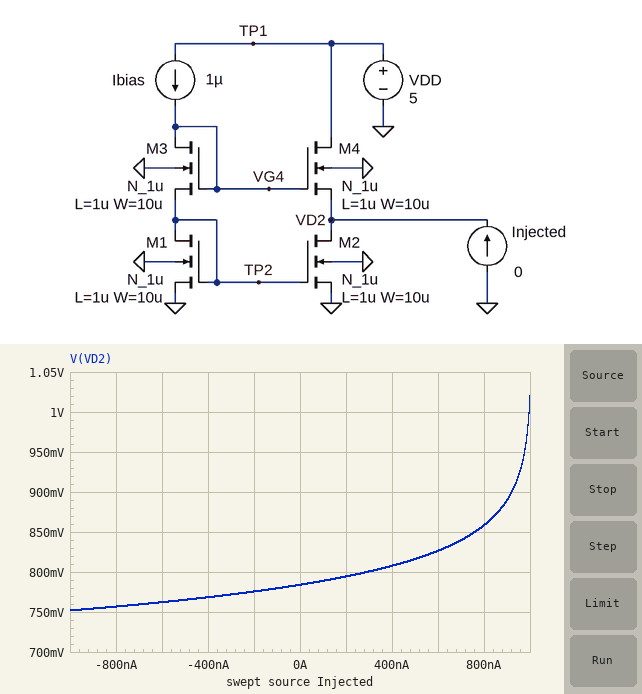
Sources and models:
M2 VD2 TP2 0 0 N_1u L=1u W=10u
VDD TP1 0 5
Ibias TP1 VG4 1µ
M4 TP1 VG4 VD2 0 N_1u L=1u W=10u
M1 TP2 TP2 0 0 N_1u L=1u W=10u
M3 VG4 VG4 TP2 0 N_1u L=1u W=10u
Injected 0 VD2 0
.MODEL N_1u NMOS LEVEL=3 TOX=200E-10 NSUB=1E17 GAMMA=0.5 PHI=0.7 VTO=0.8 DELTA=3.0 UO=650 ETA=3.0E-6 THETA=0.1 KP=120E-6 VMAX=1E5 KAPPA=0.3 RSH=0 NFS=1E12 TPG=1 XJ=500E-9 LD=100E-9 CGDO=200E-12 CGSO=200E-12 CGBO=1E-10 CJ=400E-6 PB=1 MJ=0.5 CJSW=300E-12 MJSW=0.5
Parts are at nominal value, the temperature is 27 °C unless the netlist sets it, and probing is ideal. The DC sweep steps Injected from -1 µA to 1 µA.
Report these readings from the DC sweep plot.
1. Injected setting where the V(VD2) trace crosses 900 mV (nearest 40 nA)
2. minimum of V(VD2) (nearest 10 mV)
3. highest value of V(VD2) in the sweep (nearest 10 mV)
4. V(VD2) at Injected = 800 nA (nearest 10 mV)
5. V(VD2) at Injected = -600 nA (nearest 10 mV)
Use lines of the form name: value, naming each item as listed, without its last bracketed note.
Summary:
Injected setting where the V(VD2) trace crosses 900 mV: 920 nA
minimum of V(VD2): 750 mV
highest value of V(VD2) in the sweep: 1.02 V
V(VD2) at Injected = 800 nA: 860 mV
V(VD2) at Injected = -600 nA: 760 mV
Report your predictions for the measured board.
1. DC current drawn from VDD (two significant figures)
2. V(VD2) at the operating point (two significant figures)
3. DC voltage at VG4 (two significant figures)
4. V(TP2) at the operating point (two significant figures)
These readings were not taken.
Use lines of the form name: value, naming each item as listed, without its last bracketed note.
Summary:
DC current drawn from VDD: 2.0 µA
V(VD2) at the operating point: 780 mV
DC voltage at VG4: 1.7 V
V(TP2) at the operating point: 780 mV
